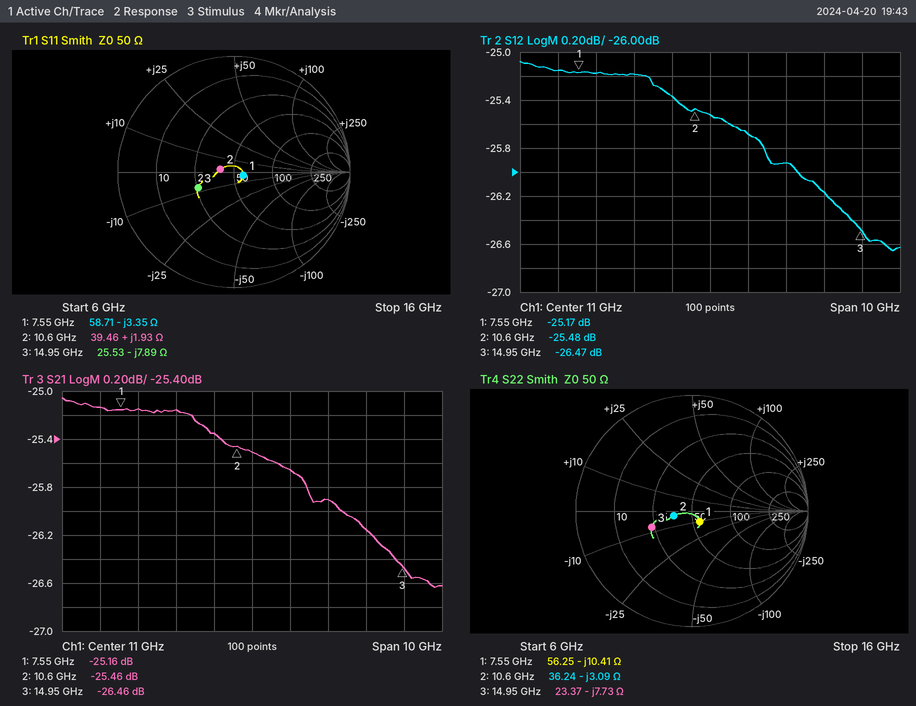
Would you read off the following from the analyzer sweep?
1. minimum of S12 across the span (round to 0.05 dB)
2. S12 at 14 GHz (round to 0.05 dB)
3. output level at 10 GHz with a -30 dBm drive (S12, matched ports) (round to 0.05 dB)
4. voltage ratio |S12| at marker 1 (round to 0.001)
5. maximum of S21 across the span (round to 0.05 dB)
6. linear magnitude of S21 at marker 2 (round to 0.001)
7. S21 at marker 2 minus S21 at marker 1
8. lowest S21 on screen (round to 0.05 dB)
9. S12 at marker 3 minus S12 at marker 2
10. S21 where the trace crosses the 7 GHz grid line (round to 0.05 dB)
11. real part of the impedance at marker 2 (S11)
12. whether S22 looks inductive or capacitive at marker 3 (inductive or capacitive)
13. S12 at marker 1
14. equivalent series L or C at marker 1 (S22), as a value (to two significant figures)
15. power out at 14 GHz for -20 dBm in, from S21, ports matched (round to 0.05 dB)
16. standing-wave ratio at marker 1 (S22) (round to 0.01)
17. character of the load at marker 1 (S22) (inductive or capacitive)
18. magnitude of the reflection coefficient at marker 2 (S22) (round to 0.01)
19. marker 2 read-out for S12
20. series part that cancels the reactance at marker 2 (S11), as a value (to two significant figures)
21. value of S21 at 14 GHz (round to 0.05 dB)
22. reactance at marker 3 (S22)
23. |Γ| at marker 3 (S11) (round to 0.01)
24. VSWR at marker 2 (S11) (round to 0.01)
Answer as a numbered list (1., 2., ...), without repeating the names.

1. -26.65 dB
2. -26.15 dB
3. -55.35 dBm
4. 0.055
5. -25.05 dB
6. 0.053
7. -0.30 dB
8. -26.65 dB
9. -0.99 dB
10. -25.15 dB
11. 39.46 Ω
12. capacitive
13. -25.17 dB
14. 2.0 pF
15. -46.15 dBm
16. 1.26
17. capacitive
18. 0.16
19. -25.48 dB
20. 7.8 pF
21. -26.15 dB
22. -7.73 Ω
23. 0.34
24. 1.27
